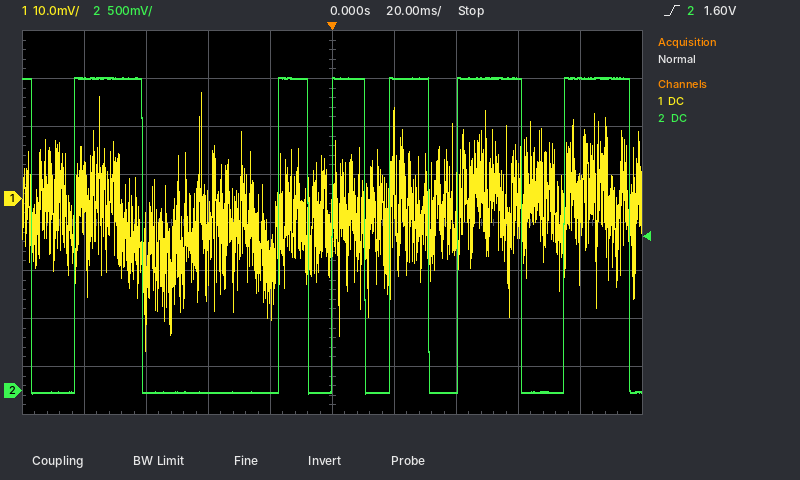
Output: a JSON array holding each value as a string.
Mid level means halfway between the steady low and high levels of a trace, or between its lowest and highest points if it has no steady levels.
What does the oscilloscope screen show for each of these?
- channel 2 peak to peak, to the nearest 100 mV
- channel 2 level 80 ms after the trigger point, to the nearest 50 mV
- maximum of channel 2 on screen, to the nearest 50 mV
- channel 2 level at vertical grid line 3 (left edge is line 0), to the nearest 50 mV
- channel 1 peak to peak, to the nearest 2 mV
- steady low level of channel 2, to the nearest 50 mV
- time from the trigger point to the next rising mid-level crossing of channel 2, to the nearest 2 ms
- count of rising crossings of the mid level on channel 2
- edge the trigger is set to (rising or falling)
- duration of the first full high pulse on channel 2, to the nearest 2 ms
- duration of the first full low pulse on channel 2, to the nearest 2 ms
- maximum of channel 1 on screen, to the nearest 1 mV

["3.30 V", "3.25 V", "3.25 V", "0 mV", "54 mV", "0 mV", "18 ms", "6", "rising", "22 ms", "14 ms", "22 mV"]
